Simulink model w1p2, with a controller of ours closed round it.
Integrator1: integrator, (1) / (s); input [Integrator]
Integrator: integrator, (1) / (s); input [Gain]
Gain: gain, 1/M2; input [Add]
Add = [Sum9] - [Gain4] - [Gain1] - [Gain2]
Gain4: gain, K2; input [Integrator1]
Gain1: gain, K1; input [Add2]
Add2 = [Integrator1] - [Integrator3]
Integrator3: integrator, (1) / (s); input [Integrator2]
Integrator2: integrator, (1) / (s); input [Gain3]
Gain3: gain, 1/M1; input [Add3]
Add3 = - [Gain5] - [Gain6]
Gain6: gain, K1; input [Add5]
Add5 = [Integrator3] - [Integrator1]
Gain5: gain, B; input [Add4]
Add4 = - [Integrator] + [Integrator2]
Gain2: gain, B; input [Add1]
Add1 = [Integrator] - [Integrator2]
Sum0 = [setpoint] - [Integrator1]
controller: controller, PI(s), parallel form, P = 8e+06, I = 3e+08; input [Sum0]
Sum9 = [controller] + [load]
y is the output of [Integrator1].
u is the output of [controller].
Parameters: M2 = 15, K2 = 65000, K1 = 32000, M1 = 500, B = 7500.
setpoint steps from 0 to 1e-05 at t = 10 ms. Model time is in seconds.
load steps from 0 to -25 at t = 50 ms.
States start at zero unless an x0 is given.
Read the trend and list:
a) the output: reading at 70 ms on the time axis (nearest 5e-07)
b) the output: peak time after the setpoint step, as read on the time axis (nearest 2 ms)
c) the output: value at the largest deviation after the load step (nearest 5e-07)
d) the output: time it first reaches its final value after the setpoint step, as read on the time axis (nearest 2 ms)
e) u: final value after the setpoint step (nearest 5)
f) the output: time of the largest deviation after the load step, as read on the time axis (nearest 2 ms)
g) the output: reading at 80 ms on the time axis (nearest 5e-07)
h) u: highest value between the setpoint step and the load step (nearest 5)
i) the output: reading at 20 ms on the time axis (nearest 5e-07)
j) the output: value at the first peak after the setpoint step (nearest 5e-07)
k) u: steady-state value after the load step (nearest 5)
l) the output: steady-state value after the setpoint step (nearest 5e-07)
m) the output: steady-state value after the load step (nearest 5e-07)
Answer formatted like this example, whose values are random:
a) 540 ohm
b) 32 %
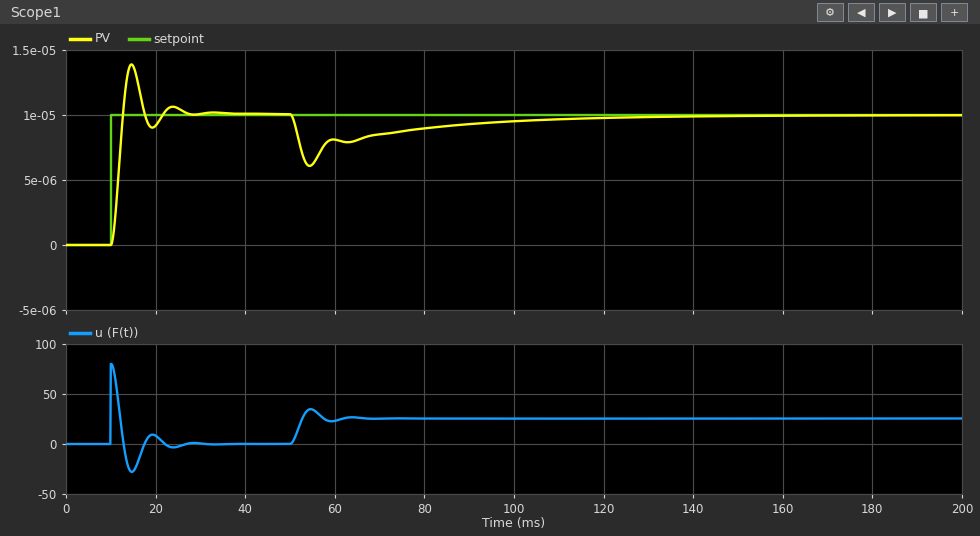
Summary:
a) 0.0000085
b) 14 ms
c) 0.0000060
d) 12 ms
e) 0
f) 54 ms
g) 0.0000090
h) 80
i) 0.0000090
j) 0.0000140
k) 25
l) 0.0000100
m) 0.0000100
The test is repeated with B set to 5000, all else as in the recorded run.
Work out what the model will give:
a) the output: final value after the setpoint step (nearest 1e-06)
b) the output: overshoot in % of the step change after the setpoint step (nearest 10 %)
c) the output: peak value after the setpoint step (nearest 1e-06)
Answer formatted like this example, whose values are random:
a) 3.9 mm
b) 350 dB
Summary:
a) 0.000010
b) 50 %
c) 0.000015
